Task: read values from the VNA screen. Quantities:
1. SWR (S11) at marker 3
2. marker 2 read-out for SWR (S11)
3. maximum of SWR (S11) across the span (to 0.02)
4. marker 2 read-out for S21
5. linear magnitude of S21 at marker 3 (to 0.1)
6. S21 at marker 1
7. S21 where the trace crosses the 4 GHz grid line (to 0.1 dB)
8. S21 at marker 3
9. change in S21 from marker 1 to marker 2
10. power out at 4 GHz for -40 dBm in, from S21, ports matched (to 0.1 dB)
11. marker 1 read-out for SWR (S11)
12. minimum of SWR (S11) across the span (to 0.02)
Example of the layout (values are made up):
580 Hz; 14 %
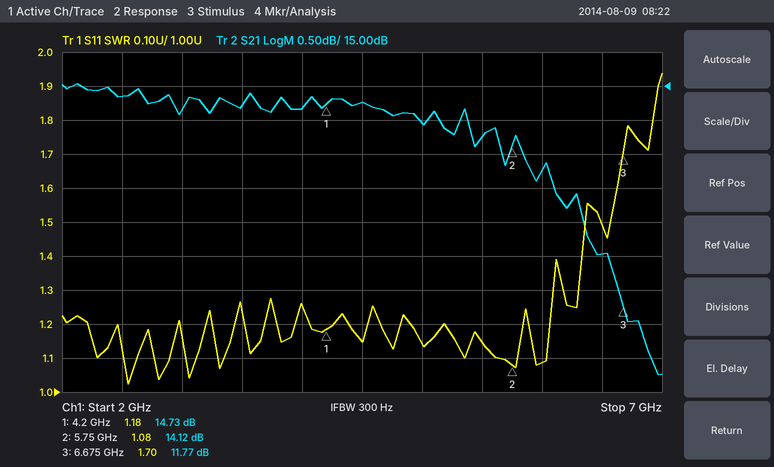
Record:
1.70; 1.08; 1.94; 14.12 dB; 3.9; 14.73 dB; 14.7 dB; 11.77 dB; -0.61 dB; -25.3 dBm; 1.18; 1.02
